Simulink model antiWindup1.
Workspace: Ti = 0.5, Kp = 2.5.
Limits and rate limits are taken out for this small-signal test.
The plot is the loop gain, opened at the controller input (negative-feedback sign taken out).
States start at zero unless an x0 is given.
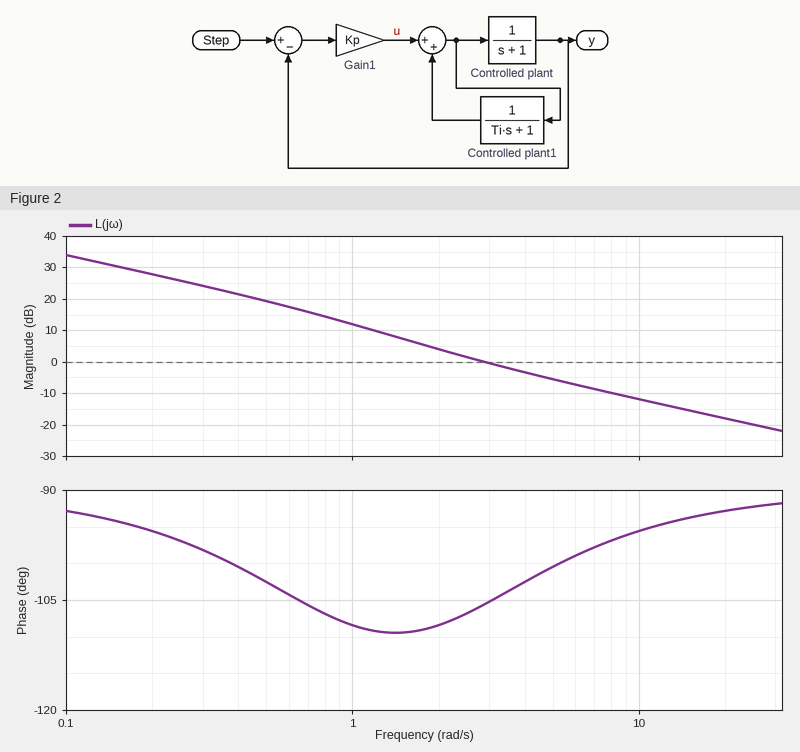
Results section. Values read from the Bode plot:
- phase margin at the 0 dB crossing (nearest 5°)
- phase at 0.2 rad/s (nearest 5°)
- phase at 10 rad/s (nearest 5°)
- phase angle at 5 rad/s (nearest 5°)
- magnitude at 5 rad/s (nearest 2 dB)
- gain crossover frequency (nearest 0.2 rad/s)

75°
-95°
-95°
-100°
-6 dB
2.8 rad/s
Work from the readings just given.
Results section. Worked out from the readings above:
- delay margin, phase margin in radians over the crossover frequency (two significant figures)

0.47 s
